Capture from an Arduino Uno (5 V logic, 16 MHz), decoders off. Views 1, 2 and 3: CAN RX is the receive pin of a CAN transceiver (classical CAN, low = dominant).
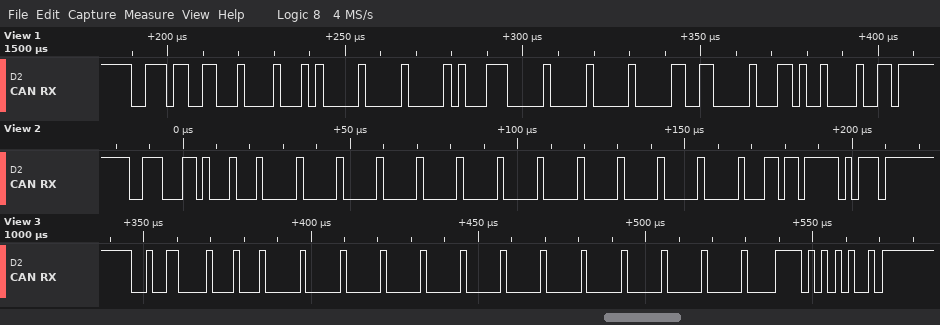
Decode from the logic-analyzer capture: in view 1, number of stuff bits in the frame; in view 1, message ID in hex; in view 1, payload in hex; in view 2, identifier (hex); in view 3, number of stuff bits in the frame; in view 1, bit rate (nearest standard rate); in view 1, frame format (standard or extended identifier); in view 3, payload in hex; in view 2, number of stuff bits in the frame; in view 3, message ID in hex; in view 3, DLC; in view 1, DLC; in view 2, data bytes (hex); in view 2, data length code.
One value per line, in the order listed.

8
0x3B3
45 00 00 8E 00 00 13 00
0x38D
12
500 kbit/s
standard
80 00 00 00 00 00 00 00
13
0x261
8
8
80 00 00 00 00 00 00 00
8
